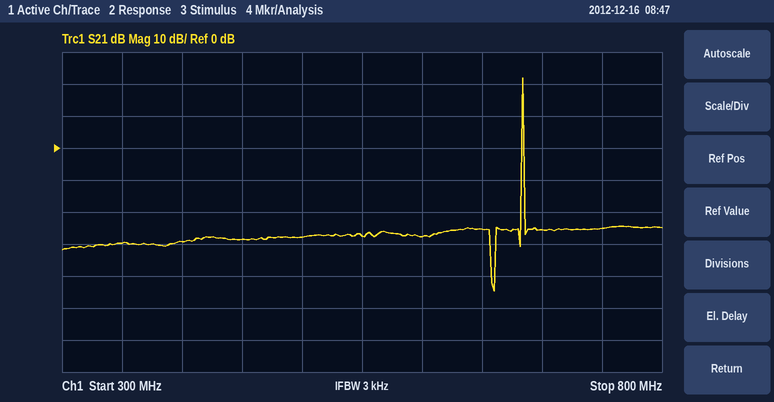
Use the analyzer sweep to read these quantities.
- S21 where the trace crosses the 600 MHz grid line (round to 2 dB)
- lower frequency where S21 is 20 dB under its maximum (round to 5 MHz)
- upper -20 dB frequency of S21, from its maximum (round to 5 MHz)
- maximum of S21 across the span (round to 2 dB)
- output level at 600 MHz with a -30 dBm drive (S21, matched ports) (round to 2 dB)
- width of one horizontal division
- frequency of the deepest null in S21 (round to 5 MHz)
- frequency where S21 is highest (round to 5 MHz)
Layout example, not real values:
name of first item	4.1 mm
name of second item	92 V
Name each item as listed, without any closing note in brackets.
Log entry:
S21 where the trace crosses the 600 MHz grid line	-28 dB
lower frequency where S21 is 20 dB under its maximum	685 MHz
upper -20 dB frequency of S21, from its maximum	685 MHz
maximum of S21 across the span	22 dB
output level at 600 MHz with a -30 dBm drive (S21, matched ports)	-58 dBm
width of one horizontal division	50 MHz
frequency of the deepest null in S21	660 MHz
frequency where S21 is highest	685 MHz
